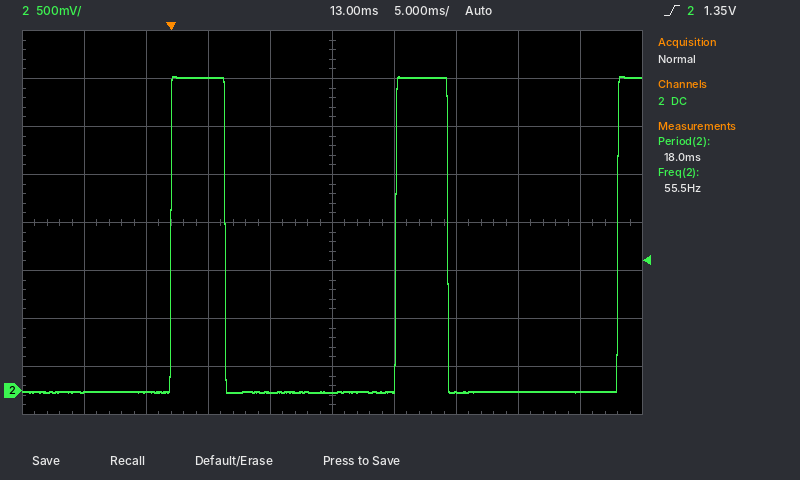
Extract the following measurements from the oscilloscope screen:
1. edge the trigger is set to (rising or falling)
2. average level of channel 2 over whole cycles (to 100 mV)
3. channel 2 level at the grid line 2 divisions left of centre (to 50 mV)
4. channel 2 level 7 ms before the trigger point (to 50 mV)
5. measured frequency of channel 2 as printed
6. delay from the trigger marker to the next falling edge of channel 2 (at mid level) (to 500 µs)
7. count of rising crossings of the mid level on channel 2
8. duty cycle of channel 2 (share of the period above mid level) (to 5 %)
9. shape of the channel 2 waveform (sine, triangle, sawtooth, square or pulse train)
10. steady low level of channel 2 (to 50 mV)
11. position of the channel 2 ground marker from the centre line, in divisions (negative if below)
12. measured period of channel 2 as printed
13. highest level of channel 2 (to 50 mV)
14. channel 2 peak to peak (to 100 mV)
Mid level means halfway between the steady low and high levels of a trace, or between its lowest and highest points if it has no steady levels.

rising
800 mV
3.25 V
0 mV
55.5 Hz
4.5 ms
3
25 %
pulse train
0 mV
-3.5 div
18.0 ms
3.25 V
3.30 V
